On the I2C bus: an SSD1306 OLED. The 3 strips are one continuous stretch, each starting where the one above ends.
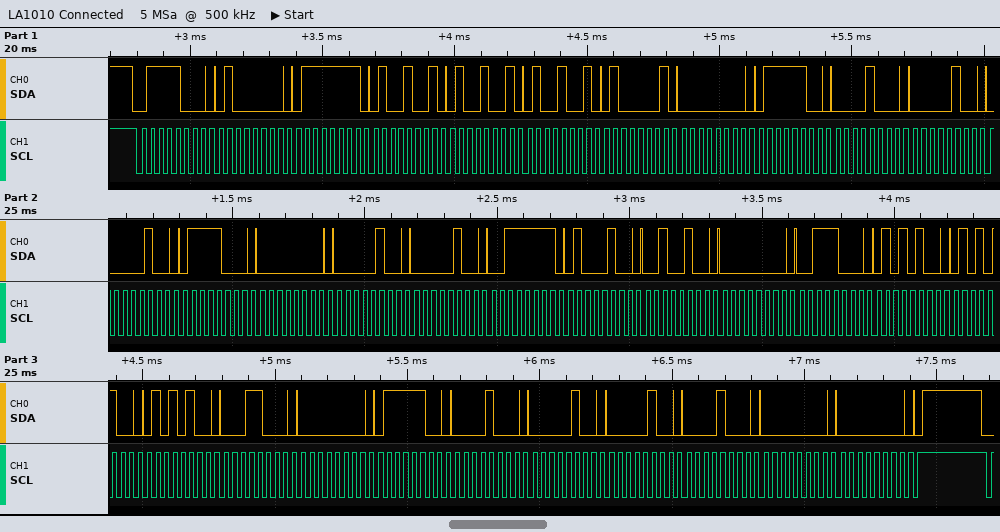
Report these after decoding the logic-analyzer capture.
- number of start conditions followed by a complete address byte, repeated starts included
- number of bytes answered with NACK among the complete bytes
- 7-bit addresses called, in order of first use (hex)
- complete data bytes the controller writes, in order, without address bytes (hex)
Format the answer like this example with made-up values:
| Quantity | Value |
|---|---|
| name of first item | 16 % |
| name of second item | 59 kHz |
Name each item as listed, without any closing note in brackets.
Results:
| Quantity | Value |
|---|---|
| number of start conditions followed by a complete address byte, repeated starts included | 1 |
| number of bytes answered with NACK among the complete bytes | 0 |
| 7-bit addresses called, in order of first use | 0x3C |
| complete data bytes the controller writes, in order, without address bytes | 40 7F 49 49 49 41 00 7C 08 04 04 78 00 04 04 3F 44 24 00 38 54 54 54 18 00 7C 08 04 04 08 00 00 |
